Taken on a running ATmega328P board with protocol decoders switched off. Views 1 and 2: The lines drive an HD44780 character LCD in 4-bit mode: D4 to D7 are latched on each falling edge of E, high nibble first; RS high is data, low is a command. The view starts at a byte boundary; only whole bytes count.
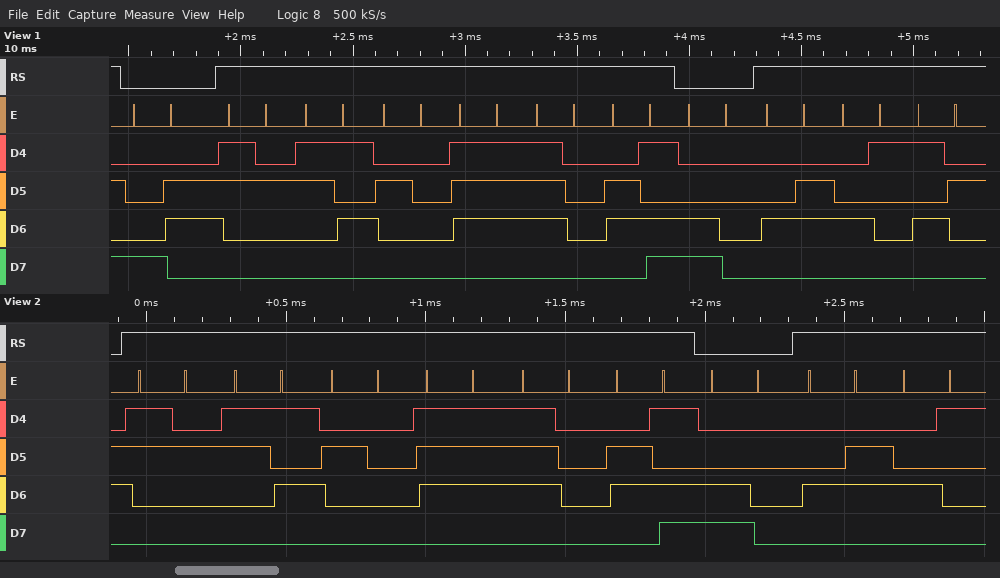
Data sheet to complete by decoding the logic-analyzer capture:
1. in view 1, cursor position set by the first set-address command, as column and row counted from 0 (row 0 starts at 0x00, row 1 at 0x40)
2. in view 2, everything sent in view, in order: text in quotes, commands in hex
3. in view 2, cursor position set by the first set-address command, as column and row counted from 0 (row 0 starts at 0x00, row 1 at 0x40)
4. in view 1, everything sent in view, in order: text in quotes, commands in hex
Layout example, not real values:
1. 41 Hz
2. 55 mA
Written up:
1. column 6, row 0
2. "25 wpm" 0xC0 "FA"
3. column 0, row 1
4. 0x86 "25 wpm" 0xC0 "FAR"
